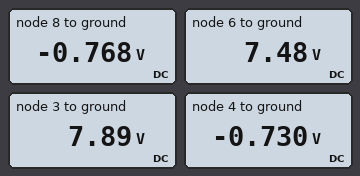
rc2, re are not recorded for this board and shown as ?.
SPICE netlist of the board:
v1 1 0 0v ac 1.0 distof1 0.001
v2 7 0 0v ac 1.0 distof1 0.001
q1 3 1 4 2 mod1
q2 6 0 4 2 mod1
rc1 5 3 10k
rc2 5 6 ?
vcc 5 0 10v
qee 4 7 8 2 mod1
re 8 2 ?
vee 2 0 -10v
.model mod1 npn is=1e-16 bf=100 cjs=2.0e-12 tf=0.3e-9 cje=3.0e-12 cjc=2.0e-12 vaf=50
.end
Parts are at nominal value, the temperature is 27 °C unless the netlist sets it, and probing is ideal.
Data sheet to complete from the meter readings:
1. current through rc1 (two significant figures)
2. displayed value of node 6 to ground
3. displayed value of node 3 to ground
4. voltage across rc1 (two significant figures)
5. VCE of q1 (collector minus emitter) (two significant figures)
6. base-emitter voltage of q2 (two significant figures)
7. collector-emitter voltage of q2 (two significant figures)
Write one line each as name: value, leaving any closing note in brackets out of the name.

current through rc1: 210 µA
displayed value of node 6 to ground: 7.48 V
displayed value of node 3 to ground: 7.89 V
voltage across rc1: 2.1 V
VCE of q1 (collector minus emitter): 8.6 V
base-emitter voltage of q2: 730 mV
collector-emitter voltage of q2: 8.2 V
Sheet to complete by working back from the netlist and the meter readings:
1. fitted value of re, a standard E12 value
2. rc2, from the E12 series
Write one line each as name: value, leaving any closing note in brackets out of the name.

fitted value of re, a standard E12 value: 15 kΩ
rc2, from the E12 series: 12 kΩ
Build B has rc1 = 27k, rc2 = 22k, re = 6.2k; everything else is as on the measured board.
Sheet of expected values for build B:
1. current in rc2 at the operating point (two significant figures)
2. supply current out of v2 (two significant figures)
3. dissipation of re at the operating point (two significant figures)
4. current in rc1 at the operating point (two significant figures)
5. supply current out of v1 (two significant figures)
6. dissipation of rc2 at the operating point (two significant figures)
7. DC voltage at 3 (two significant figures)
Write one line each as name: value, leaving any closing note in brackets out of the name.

current in rc2 at the operating point: 480 µA
supply current out of v2: 530 µA
dissipation of re at the operating point: 14 mW
current in rc1 at the operating point: 400 µA
supply current out of v1: 59 µA
dissipation of rc2 at the operating point: 5.2 mW
DC voltage at 3: -700 mV
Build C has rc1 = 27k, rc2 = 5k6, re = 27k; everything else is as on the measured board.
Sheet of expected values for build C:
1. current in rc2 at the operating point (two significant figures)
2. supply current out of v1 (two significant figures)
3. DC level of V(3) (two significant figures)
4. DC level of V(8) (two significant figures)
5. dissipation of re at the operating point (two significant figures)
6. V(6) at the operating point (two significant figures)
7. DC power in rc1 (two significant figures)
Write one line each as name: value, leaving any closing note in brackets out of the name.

current in rc2 at the operating point: 120 µA
supply current out of v1: 1.0 µA
DC level of V(3): 6.9 V
DC level of V(8): -750 mV
dissipation of re at the operating point: 3.2 mW
V(6) at the operating point: 9.3 V
DC power in rc1: 360 µW
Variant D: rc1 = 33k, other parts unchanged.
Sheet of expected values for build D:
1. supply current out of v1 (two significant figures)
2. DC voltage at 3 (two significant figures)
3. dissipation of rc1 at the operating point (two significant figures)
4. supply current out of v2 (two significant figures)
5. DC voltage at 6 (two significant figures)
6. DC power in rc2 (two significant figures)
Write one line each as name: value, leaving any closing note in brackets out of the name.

supply current out of v1: 1.9 µA
DC voltage at 3: 3.4 V
dissipation of rc1 at the operating point: 1.3 mW
supply current out of v2: 200 µA
DC voltage at 6: 7.4 V
DC power in rc2: 560 µW
